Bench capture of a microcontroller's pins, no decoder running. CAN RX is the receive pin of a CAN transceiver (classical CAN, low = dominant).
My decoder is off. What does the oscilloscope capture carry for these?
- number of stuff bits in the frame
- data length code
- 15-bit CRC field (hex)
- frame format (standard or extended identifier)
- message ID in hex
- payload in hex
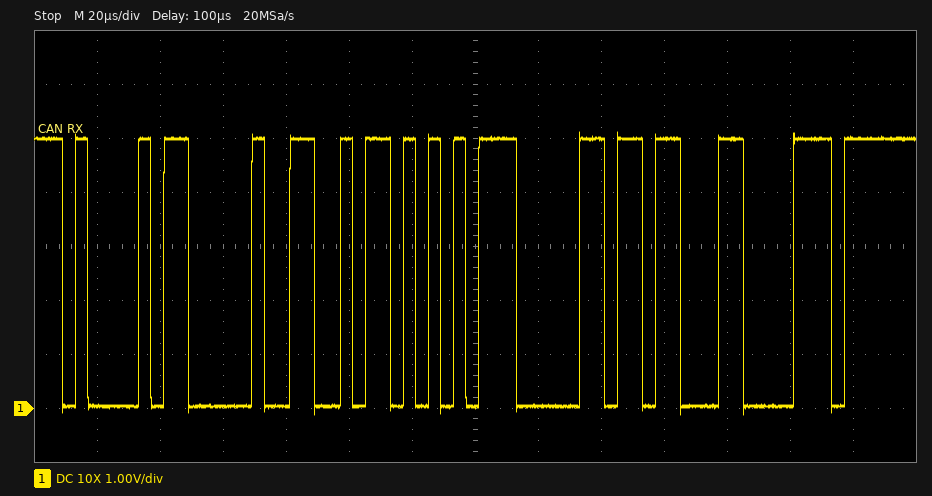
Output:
2
3
0x58C3
standard
0x42C
2D 57 05
